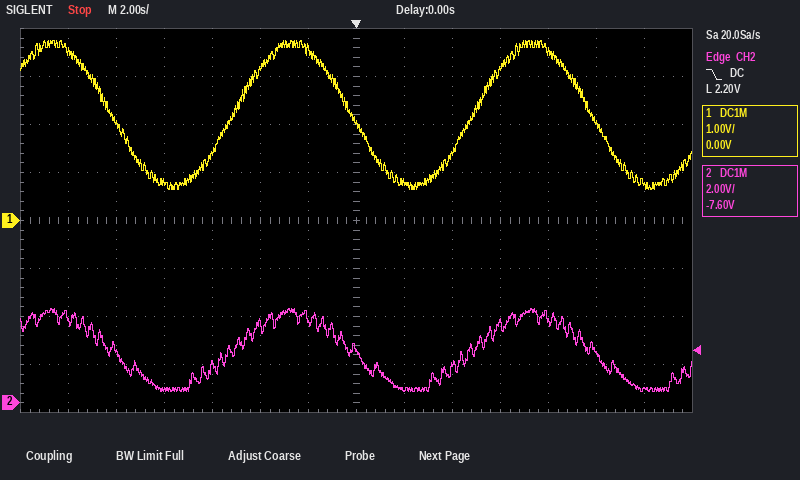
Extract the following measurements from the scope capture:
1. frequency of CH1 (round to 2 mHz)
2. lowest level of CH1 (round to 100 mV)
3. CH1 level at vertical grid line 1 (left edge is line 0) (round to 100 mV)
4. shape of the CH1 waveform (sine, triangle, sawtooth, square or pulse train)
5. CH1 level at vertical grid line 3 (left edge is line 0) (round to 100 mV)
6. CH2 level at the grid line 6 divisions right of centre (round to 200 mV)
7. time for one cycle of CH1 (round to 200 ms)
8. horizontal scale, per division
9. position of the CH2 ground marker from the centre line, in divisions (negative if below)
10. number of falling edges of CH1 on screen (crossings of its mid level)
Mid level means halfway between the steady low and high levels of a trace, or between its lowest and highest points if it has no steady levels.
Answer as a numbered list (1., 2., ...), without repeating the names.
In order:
1. 100 mHz
2. 600 mV
3. 3.5 V
4. sine
5. 800 mV
6. 600 mV
7. 10.0 s
8. 2 s
9. -3.8 div
10. 3
